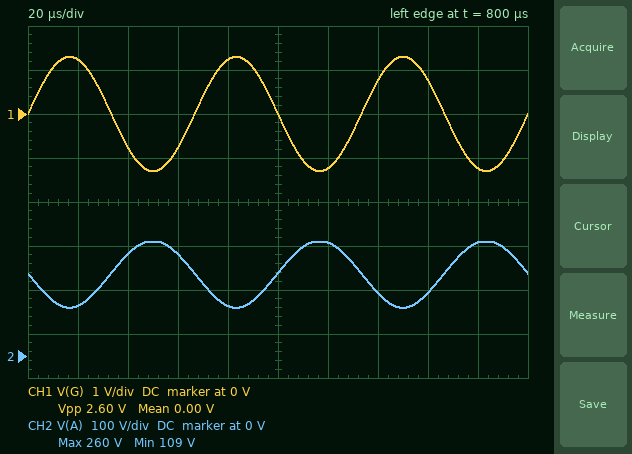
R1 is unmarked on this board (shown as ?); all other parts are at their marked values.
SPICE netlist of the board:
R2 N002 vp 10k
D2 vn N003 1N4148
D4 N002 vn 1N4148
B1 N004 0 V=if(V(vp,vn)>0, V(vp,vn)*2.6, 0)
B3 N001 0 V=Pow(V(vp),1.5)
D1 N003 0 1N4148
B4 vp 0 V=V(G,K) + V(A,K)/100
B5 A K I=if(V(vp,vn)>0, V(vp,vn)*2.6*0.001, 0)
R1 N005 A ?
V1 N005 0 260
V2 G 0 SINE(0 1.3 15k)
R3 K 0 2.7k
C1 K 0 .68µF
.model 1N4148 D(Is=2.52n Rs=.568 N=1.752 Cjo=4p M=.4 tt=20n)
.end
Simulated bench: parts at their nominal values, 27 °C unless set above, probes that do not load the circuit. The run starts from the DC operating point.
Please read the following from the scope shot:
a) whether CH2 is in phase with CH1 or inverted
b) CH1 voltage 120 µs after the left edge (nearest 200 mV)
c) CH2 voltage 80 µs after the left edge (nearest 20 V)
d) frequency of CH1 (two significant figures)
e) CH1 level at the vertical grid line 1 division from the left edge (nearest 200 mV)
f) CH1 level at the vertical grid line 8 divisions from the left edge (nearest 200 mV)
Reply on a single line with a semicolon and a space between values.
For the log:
inverted; -1.2 V; 120 V; 15 kHz; 1.2 V; 800 mV
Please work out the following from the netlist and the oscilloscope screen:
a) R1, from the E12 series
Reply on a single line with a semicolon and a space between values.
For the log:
150 kΩ
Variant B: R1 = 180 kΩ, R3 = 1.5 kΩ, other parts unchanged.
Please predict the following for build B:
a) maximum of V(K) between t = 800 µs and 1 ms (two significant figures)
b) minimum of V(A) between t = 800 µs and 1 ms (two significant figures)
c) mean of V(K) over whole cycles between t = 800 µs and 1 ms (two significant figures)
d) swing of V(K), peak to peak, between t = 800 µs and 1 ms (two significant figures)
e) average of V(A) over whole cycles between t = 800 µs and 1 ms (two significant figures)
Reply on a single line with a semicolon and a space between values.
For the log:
890 mV; 70 V; 880 mV; 14 mV; 150 V
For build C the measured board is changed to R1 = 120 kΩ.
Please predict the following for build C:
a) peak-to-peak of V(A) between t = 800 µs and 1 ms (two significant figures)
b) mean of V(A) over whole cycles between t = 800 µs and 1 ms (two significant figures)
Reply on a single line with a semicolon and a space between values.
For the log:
130 V; 200 V
